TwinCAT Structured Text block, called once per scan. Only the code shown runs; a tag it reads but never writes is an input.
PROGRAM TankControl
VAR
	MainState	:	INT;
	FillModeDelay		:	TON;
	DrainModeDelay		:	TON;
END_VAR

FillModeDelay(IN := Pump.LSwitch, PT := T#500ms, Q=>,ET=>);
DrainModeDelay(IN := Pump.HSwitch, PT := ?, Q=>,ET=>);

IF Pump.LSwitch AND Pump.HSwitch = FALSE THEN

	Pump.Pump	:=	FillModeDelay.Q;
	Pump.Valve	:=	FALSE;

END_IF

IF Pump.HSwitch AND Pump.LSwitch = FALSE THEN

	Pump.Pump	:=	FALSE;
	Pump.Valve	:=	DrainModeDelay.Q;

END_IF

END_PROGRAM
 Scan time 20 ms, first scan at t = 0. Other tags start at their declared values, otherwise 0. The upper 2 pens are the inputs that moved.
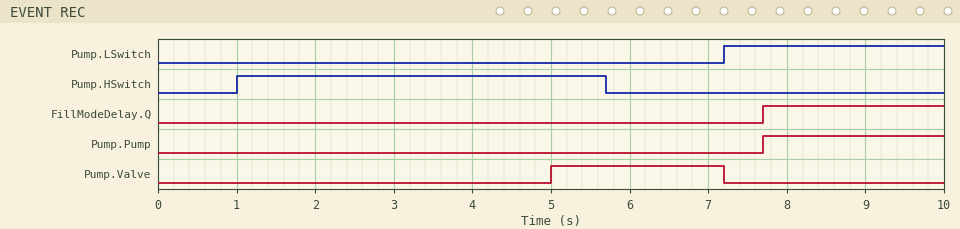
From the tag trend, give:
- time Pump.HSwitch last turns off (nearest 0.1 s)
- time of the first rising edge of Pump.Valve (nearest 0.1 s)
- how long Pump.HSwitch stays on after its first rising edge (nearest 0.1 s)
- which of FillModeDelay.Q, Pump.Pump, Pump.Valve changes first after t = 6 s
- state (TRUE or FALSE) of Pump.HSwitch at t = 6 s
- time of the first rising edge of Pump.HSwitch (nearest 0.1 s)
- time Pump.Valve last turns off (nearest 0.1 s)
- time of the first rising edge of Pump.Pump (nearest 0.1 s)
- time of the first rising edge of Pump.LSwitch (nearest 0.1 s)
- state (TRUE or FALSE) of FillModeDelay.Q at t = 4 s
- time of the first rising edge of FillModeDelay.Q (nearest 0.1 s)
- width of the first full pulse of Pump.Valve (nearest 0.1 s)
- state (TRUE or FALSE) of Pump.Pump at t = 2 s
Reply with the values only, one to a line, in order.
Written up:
5.7 s
5.0 s
4.7 s
Pump.Valve
FALSE
1.0 s
7.2 s
7.7 s
7.2 s
FALSE
7.7 s
2.2 s
FALSE
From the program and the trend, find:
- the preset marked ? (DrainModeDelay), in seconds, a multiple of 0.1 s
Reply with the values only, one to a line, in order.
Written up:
4.0 s
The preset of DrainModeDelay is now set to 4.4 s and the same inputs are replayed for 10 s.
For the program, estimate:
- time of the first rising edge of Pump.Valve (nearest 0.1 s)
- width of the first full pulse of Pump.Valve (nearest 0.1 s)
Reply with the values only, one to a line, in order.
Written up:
5.4 s
1.8 s
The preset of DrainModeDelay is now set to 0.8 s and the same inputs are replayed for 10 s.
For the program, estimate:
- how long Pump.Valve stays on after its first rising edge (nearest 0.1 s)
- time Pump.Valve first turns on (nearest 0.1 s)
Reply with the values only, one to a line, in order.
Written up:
5.4 s
1.8 s
